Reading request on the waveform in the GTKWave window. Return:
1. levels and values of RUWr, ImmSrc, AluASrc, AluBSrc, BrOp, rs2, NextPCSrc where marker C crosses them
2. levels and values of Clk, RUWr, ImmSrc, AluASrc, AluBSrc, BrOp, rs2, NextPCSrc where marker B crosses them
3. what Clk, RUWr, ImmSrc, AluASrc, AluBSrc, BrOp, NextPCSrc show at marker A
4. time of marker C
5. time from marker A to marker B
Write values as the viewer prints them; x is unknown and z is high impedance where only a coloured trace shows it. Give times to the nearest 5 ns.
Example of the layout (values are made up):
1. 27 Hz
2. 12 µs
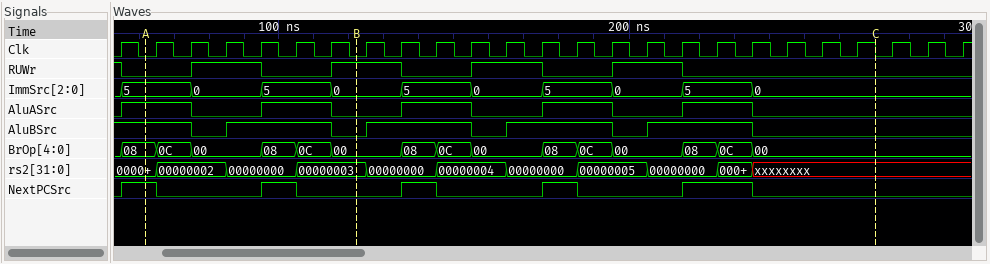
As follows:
1. RUWr=0, ImmSrc=0, AluASrc=0, AluBSrc=0, BrOp=00, rs2=xxxxxxxx, NextPCSrc=0
2. Clk=0, RUWr=1, ImmSrc=0, AluASrc=0, AluBSrc=0, BrOp=00, rs2=00000003, NextPCSrc=0
3. Clk=0, RUWr=0, ImmSrc=5, AluASrc=1, AluBSrc=1, BrOp=08, NextPCSrc=1
4. 270 ns
5. 60 ns
